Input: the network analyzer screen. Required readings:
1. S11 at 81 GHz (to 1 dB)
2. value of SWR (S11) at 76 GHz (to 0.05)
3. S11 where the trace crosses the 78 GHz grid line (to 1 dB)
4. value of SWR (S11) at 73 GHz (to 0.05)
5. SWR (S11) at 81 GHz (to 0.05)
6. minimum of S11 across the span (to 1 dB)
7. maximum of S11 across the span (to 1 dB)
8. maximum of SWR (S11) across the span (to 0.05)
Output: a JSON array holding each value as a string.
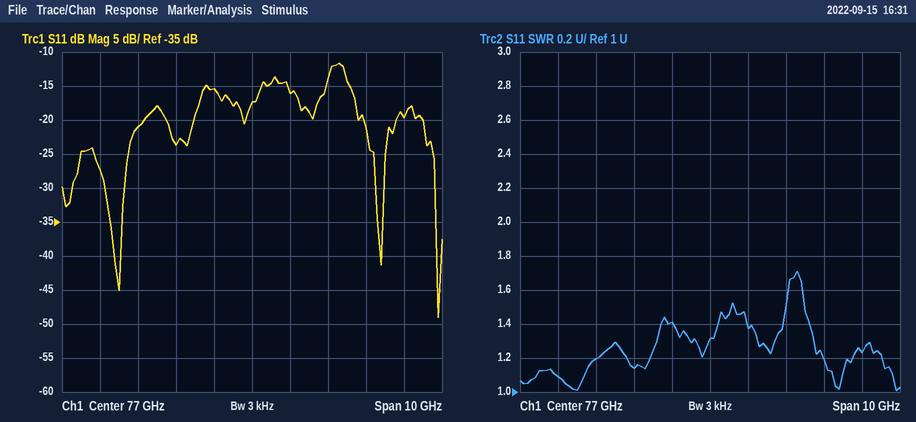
["-20 dB", "1.40", "-16 dB", "1.10", "1.25", "-49 dB", "-12 dB", "1.70"]
